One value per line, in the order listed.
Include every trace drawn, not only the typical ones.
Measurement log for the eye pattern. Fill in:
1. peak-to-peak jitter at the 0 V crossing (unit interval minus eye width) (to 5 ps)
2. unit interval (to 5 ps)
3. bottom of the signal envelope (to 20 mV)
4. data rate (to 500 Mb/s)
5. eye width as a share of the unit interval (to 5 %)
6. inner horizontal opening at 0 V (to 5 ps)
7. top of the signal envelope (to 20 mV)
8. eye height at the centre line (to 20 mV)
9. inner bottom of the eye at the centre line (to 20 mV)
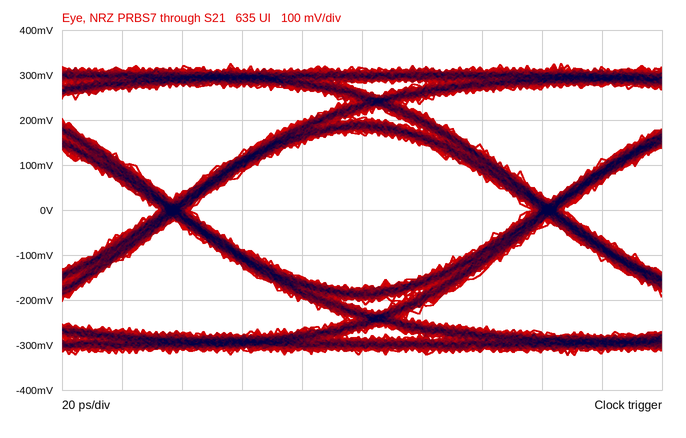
10 ps
125 ps
-320 mV
8.0 Gb/s
90 %
115 ps
320 mV
340 mV
-180 mV
